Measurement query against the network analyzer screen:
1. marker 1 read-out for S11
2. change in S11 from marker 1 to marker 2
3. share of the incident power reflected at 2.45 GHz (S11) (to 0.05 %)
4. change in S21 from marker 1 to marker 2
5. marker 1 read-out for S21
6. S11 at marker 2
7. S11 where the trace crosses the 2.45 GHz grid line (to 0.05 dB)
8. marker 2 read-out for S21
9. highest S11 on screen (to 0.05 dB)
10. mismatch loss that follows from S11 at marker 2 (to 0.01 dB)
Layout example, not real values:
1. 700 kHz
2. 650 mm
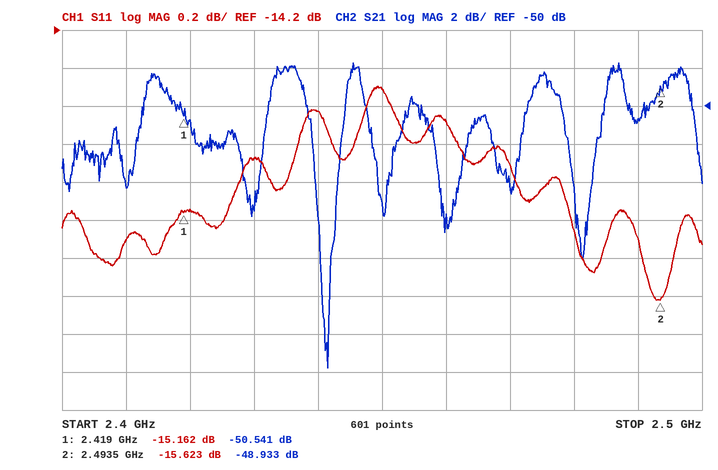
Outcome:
1. -15.162 dB
2. -0.461 dB
3. 3.55 %
4. 1.608 dB
5. -50.541 dB
6. -15.623 dB
7. -14.50 dB
8. -48.933 dB
9. -14.50 dB
10. 0.12 dB
